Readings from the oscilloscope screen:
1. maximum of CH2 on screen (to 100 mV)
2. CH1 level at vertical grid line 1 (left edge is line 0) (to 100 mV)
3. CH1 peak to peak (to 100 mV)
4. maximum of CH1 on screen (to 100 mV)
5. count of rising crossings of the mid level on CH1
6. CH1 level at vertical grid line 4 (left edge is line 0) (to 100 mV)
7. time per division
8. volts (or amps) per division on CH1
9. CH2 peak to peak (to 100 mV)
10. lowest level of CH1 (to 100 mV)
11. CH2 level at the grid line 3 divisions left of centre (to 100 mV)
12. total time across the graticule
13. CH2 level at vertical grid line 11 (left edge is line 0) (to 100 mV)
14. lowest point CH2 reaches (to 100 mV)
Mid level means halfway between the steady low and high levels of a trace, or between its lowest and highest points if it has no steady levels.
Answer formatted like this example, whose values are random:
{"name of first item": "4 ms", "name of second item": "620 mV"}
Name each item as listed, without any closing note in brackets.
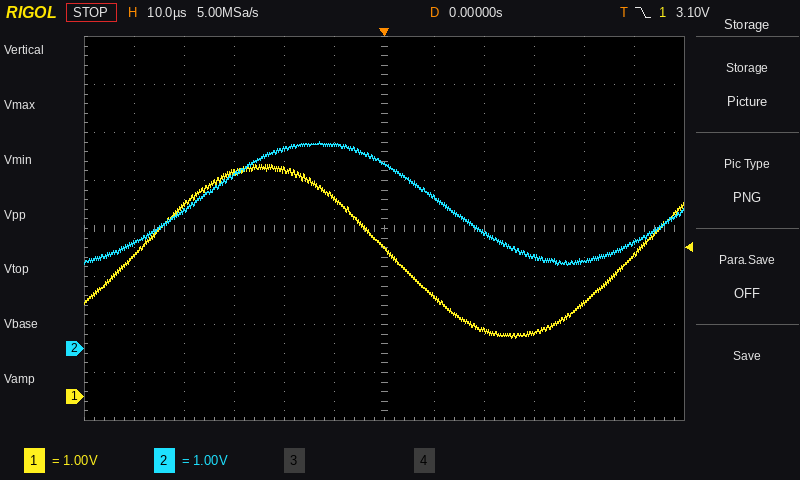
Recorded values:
{"maximum of CH2 on screen": "4.3 V", "CH1 level at vertical grid line 1 (left edge is line 0)": "2.9 V", "CH1 peak to peak": "3.6 V", "maximum of CH1 on screen": "4.8 V", "count of rising crossings of the mid level on CH1": "2", "CH1 level at vertical grid line 4 (left edge is line 0)": "4.7 V", "time per division": "10 µs", "volts (or amps) per division on CH1": "1 V", "CH2 peak to peak": "2.6 V", "lowest level of CH1": "1.2 V", "CH2 level at the grid line 3 divisions left of centre": "3.6 V", "total time across the graticule": "120 µs", "CH2 level at vertical grid line 11 (left edge is line 0)": "2.2 V", "lowest point CH2 reaches": "1.7 V"}
